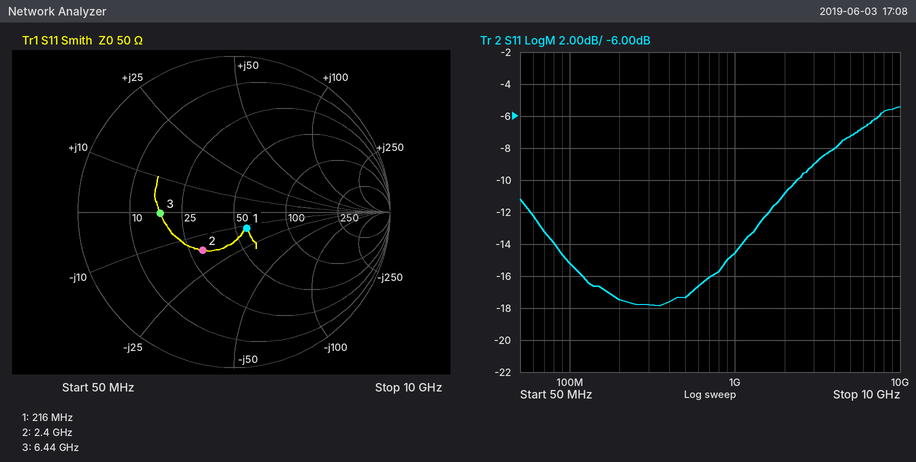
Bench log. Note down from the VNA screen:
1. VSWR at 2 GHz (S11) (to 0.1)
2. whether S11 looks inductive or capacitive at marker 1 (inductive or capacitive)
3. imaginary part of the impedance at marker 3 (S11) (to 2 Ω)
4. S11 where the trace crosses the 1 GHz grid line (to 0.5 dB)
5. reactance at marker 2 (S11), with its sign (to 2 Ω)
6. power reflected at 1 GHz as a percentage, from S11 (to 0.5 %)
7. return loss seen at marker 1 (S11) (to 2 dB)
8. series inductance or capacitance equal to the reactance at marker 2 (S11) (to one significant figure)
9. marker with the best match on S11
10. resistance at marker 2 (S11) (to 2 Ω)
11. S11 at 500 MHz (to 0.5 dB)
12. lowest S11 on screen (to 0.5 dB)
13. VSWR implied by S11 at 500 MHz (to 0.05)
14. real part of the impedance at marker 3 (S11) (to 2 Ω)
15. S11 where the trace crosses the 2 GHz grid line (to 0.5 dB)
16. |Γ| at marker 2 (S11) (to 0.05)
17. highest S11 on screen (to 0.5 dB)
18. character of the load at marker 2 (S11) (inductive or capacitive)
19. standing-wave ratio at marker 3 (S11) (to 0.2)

1.8
capacitive
0 Ω
-14.5 dB
-16 Ω
3.5 %
18 dB
4 pF
marker 1
30 Ω
-17.5 dB
-18.0 dB
1.30
18 Ω
-11.0 dB
0.30
-5.5 dB
capacitive
2.8
